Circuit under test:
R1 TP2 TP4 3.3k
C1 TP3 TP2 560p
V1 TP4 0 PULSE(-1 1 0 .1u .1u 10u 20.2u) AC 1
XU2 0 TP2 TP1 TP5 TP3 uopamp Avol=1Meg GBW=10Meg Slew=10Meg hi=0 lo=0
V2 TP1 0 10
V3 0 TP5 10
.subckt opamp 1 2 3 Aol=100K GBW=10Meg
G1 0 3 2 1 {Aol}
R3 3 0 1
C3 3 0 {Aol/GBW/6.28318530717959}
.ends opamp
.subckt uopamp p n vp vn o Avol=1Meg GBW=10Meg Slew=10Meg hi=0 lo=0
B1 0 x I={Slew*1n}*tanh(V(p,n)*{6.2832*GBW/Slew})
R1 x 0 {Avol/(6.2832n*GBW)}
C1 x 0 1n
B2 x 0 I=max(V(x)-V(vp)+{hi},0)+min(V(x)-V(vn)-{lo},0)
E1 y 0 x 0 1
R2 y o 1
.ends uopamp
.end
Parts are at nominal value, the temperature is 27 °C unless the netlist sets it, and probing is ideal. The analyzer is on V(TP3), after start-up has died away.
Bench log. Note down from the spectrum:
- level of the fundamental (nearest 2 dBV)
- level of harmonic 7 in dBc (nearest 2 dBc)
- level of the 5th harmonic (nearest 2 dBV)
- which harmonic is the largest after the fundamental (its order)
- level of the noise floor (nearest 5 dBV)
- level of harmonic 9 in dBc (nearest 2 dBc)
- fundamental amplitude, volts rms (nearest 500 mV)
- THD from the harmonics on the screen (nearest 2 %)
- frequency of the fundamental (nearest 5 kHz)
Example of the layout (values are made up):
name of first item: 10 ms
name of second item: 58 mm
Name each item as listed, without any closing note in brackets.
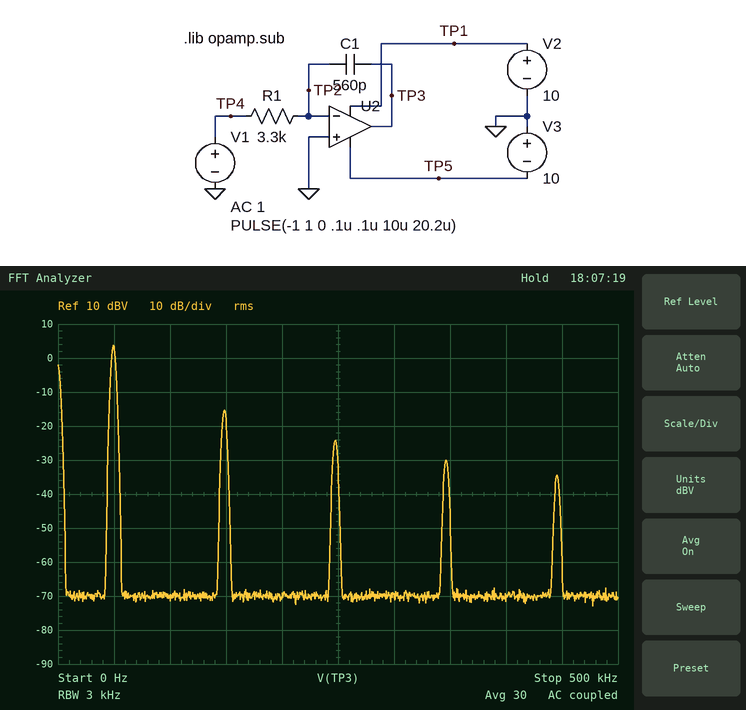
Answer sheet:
level of the fundamental: 4 dBV
level of harmonic 7 in dBc: -34 dBc
level of the 5th harmonic: -24 dBV
which harmonic is the largest after the fundamental: 3
level of the noise floor: -70 dBV
level of harmonic 9 in dBc: -38 dBc
fundamental amplitude, volts rms: 1.5 V
THD from the harmonics on the screen: 12 %
frequency of the fundamental: 50 kHz
